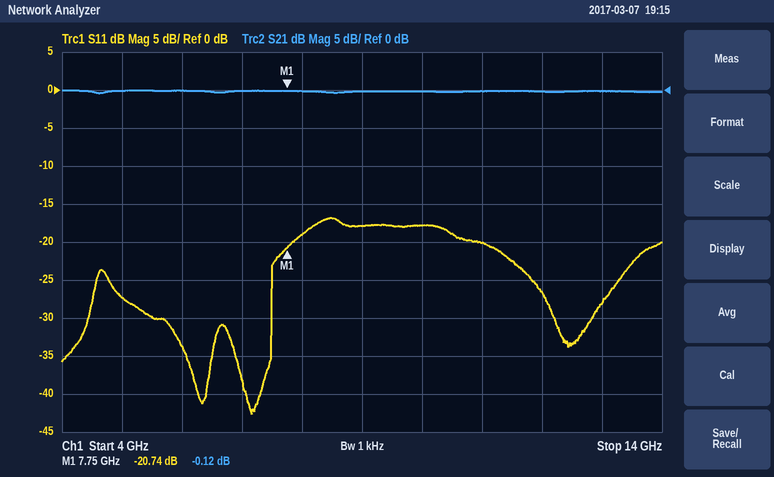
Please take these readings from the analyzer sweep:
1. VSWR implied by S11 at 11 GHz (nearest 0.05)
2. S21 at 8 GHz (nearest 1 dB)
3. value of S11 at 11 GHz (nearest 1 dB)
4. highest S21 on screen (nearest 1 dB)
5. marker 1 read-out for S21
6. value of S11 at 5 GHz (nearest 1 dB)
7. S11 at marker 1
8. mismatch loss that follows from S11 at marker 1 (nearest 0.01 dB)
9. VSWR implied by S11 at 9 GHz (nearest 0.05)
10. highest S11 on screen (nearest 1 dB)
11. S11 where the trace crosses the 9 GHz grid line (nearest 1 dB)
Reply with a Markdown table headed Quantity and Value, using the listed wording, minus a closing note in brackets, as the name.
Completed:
| Quantity | Value |
|---|---|
| VSWR implied by S11 at 11 GHz | 1.20 |
| S21 at 8 GHz | 0 dB |
| value of S11 at 11 GHz | -20 dB |
| highest S21 on screen | 0 dB |
| marker 1 read-out for S21 | -0.12 dB |
| value of S11 at 5 GHz | -27 dB |
| S11 at marker 1 | -20.74 dB |
| mismatch loss that follows from S11 at marker 1 | 0.04 dB |
| VSWR implied by S11 at 9 GHz | 1.30 |
| highest S11 on screen | -17 dB |
| S11 where the trace crosses the 9 GHz grid line | -18 dB |
